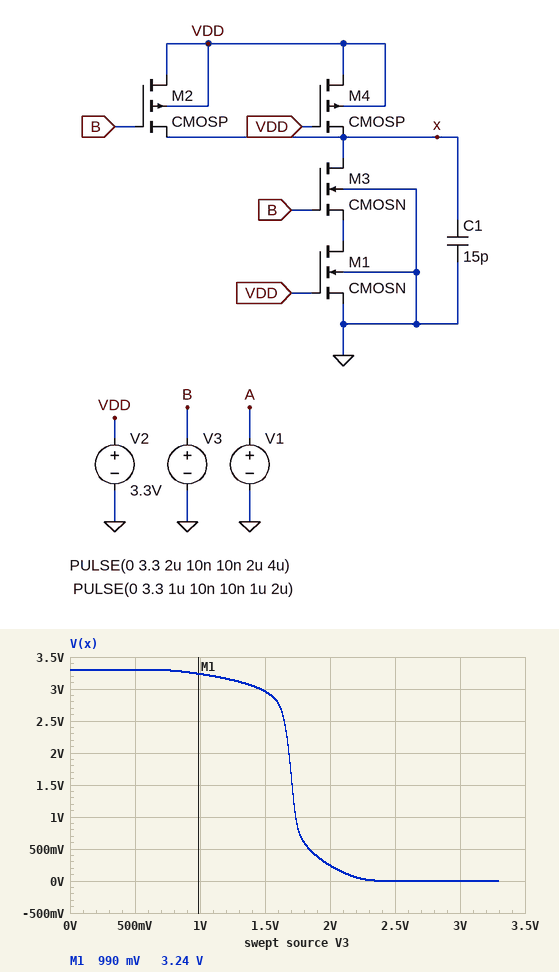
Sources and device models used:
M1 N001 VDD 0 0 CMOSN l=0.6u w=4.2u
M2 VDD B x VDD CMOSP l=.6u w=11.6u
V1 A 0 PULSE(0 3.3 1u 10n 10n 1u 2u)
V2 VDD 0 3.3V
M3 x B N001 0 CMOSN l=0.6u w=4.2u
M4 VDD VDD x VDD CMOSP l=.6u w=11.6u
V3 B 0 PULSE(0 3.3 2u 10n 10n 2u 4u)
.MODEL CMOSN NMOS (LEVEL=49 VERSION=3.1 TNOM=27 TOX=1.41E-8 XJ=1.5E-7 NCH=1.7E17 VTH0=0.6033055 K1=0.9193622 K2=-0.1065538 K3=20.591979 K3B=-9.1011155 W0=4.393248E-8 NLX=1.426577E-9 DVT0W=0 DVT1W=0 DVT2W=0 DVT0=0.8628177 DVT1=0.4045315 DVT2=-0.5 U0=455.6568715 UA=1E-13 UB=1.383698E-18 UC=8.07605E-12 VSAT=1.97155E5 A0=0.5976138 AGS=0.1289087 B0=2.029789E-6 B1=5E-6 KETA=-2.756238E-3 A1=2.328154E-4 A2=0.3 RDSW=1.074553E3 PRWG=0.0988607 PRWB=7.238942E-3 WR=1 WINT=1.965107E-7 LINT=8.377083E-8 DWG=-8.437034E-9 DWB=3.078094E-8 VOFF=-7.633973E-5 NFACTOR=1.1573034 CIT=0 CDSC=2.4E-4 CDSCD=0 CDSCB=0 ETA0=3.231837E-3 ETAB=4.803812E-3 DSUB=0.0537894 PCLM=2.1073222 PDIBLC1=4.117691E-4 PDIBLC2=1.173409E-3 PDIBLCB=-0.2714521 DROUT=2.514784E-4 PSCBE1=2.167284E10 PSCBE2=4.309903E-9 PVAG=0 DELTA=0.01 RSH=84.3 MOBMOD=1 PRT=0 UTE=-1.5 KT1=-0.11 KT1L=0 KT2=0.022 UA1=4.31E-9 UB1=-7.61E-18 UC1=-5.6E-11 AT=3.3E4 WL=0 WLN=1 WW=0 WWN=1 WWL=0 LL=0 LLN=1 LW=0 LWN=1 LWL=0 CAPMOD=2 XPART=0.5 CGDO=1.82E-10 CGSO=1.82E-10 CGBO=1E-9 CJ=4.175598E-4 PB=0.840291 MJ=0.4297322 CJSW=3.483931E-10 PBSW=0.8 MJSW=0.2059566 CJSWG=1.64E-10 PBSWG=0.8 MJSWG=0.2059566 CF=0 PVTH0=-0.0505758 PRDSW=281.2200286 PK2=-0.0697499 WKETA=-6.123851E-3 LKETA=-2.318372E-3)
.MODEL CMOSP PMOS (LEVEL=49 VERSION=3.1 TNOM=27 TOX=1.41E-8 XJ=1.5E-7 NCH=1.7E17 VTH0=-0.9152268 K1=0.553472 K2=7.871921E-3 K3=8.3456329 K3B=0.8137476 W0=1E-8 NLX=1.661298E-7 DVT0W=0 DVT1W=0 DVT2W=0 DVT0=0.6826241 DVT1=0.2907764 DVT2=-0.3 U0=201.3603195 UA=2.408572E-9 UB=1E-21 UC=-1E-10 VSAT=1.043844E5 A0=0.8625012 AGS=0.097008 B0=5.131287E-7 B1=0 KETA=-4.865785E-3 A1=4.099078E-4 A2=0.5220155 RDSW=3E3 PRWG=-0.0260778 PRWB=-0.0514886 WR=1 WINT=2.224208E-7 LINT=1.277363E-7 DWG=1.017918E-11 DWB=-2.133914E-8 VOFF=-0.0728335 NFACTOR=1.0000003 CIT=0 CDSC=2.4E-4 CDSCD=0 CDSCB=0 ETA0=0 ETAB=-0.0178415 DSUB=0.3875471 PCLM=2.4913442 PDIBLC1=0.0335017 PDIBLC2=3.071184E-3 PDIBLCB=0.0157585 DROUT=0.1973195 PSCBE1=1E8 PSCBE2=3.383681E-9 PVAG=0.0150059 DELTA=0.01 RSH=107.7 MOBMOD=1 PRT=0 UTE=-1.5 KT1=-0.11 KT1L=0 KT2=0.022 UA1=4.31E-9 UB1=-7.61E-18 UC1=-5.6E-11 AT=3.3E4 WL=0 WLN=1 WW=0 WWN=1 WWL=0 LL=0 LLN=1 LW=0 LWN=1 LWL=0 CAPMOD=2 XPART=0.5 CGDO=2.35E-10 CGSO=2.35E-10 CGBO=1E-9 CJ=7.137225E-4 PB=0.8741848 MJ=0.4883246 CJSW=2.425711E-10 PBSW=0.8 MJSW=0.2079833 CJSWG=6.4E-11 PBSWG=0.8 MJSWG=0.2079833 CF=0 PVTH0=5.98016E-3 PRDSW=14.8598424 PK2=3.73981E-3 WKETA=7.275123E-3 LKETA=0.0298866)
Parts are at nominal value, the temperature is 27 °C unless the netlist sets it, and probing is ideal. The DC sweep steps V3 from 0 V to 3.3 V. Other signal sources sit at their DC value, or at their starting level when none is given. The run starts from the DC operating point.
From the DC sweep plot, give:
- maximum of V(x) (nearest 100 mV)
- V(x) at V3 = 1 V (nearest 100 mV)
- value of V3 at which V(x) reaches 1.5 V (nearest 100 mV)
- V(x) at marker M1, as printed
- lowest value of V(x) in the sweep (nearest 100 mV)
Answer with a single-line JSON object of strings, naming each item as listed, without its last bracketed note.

{"maximum of V(x)": "3.3 V", "V(x) at V3 = 1 V": "3.2 V", "value of V3 at which V(x) reaches 1.5 V": "1.7 V", "V(x) at marker M1, as printed": "3.24 V", "lowest value of V(x) in the sweep": "0 V"}
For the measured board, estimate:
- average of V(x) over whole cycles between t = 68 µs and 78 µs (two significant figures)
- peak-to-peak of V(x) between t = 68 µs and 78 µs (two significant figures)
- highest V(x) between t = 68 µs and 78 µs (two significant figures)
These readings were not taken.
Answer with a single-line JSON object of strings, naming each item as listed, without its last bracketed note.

{"average of V(x) over whole cycles between t = 68 µs and 78 µs": "1.7 V", "peak-to-peak of V(x) between t = 68 µs and 78 µs": "3.3 V", "highest V(x) between t = 68 µs and 78 µs": "3.3 V"}
